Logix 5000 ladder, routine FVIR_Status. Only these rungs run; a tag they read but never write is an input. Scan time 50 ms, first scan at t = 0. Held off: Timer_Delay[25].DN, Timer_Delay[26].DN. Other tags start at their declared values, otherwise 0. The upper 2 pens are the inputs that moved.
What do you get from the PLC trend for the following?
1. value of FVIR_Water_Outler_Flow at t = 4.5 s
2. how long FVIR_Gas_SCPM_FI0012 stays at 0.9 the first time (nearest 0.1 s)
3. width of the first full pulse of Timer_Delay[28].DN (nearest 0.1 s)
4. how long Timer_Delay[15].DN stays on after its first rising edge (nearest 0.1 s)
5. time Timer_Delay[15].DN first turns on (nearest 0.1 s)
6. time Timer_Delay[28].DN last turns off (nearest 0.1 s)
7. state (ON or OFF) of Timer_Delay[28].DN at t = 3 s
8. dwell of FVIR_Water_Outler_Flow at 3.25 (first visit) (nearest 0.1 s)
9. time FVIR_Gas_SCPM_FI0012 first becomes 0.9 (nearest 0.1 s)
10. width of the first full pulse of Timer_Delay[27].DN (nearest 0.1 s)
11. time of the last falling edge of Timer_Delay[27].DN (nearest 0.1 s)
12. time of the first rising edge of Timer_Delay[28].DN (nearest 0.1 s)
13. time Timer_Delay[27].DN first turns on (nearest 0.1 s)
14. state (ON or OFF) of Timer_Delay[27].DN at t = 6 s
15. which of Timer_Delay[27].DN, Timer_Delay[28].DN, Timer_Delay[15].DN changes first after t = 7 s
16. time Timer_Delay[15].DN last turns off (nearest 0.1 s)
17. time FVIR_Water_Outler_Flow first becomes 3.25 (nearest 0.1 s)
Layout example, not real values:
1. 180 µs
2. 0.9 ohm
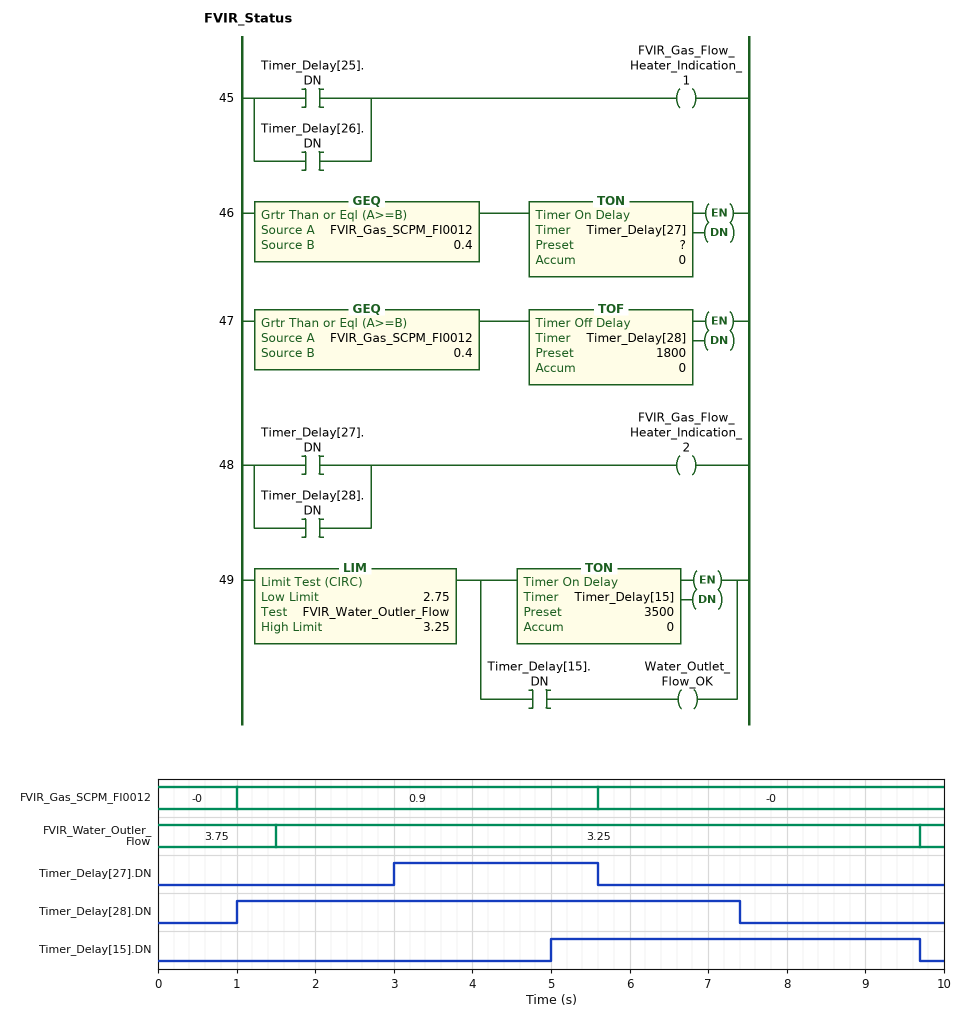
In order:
1. 3.25
2. 4.6 s
3. 6.4 s
4. 4.7 s
5. 5.0 s
6. 7.4 s
7. ON
8. 8.2 s
9. 1.0 s
10. 2.6 s
11. 5.6 s
12. 1.0 s
13. 3.0 s
14. OFF
15. Timer_Delay[28].DN
16. 9.7 s
17. 1.5 s
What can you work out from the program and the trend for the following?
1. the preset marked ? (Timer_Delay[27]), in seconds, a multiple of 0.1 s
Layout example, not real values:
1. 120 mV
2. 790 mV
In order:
1. 2.0 s
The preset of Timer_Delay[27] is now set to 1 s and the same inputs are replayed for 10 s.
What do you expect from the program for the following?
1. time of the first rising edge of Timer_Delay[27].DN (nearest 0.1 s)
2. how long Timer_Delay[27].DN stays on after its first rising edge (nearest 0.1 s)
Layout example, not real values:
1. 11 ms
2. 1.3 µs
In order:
1. 2.0 s
2. 3.6 s
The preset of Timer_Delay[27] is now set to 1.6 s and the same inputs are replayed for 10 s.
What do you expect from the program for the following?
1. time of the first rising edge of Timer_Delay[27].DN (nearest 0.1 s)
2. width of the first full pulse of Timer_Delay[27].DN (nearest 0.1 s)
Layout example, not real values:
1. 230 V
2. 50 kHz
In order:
1. 2.6 s
2. 3.0 s
